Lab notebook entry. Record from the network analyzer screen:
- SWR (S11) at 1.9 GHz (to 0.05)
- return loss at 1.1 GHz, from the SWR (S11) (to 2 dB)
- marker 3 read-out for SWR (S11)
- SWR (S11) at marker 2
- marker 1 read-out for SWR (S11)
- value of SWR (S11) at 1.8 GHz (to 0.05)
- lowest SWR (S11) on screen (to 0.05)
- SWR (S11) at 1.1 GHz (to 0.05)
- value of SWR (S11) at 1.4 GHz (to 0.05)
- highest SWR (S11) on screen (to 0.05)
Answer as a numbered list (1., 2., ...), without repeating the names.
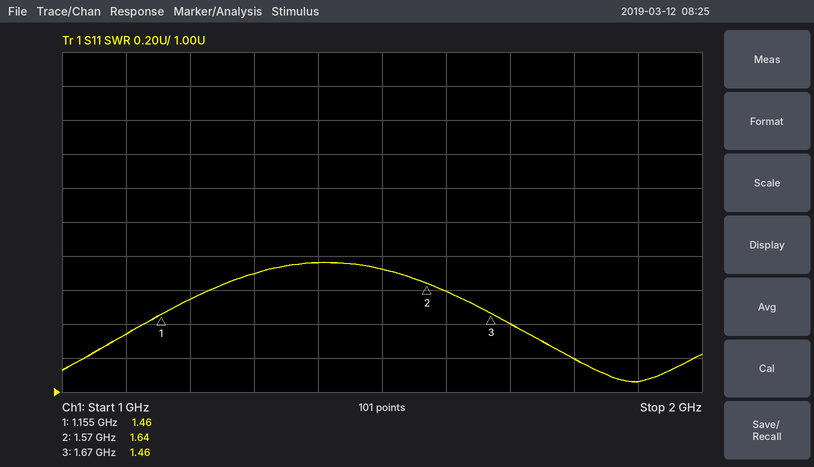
1. 1.05
2. 16 dB
3. 1.46
4. 1.64
5. 1.46
6. 1.20
7. 1.05
8. 1.35
9. 1.75
10. 1.75
